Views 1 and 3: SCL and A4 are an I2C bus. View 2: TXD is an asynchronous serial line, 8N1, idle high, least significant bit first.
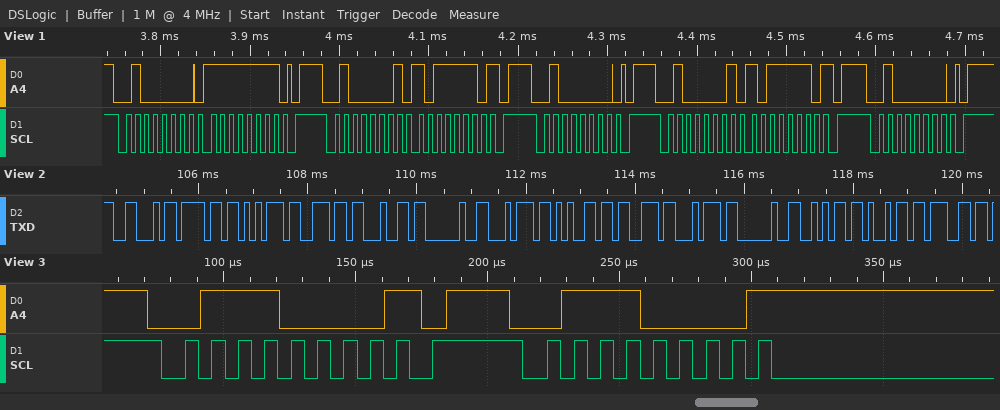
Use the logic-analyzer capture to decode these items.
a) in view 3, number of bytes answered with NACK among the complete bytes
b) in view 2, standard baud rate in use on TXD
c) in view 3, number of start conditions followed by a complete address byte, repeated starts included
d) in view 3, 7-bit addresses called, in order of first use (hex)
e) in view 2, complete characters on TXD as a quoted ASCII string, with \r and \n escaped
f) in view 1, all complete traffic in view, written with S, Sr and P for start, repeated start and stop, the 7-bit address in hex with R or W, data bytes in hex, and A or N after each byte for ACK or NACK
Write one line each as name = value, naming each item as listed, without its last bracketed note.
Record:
in view 3, number of bytes answered with NACK among the complete bytes = 2
in view 2, standard baud rate in use on TXD = 9600 baud
in view 3, number of start conditions followed by a complete address byte, repeated starts included = 2
in view 3, 7-bit addresses called, in order of first use = 0x38
in view 2, complete characters on TXD as a quoted ASCII string, with \r and \n escaped = "Found test jig"
in view 1, all complete traffic in view, written with S, Sr and P for start, repeated start and stop, the 7-bit address in hex with R or W, data bytes in hex, and A or N after each byte for ACK or NACK = S 20W A FF A P S 20R A BE N P S 20W A P S 20R A BE N P S 20W A P
